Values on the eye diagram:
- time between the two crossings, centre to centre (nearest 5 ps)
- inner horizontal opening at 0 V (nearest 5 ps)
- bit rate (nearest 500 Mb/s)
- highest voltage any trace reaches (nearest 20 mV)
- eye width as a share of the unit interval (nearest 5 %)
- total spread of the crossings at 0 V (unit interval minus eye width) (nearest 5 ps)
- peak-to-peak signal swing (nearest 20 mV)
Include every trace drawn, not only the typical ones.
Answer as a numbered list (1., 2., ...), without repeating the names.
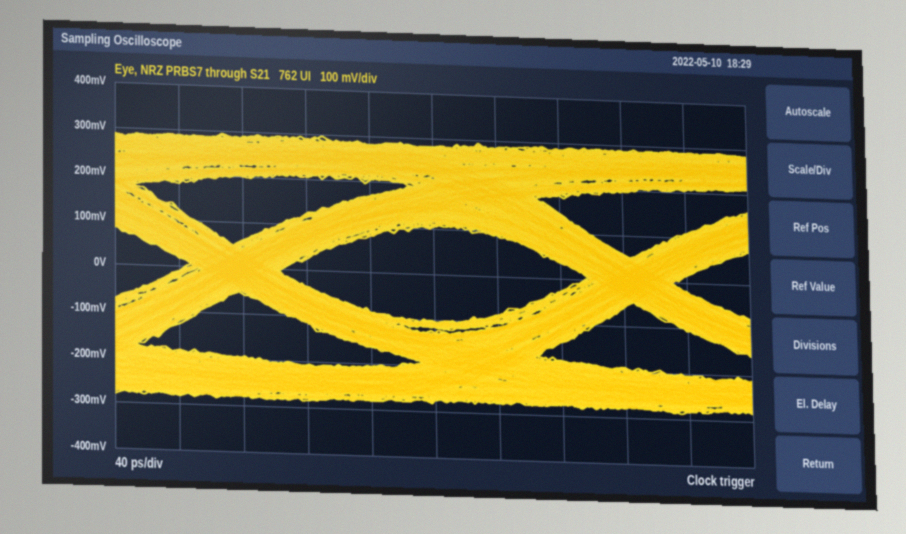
1. 250 ps
2. 190 ps
3. 4.0 Gb/s
4. 300 mV
5. 75 %
6. 60 ps
7. 580 mV
